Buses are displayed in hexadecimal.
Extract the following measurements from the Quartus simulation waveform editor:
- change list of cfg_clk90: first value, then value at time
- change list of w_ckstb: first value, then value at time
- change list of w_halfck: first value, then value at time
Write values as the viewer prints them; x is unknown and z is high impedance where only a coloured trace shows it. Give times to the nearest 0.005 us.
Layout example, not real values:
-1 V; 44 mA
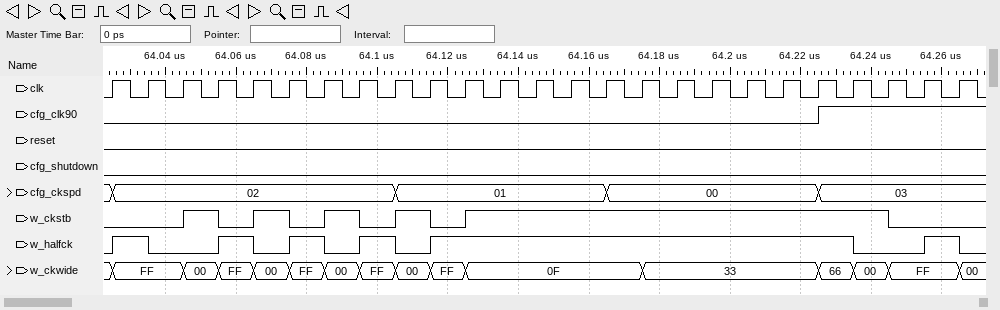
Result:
0, 1 at 64.225 us; 0, 1 at 64.045 us, 0 at 64.055 us, 1 at 64.065 us, 0 at 64.075 us, 1 at 64.085 us, 0 at 64.095 us, 1 at 64.105 us, 0 at 64.115 us, 1 at 64.125 us, 0 at 64.245 us; 0, 1 at 64.025 us, 0 at 64.035 us, 1 at 64.055 us, 0 at 64.065 us, 1 at 64.075 us, 0 at 64.085 us, 1 at 64.095 us, 0 at 64.105 us, 1 at 64.115 us, 0 at 64.235 us, 1 at 64.255 us, 0 at 64.265 us
